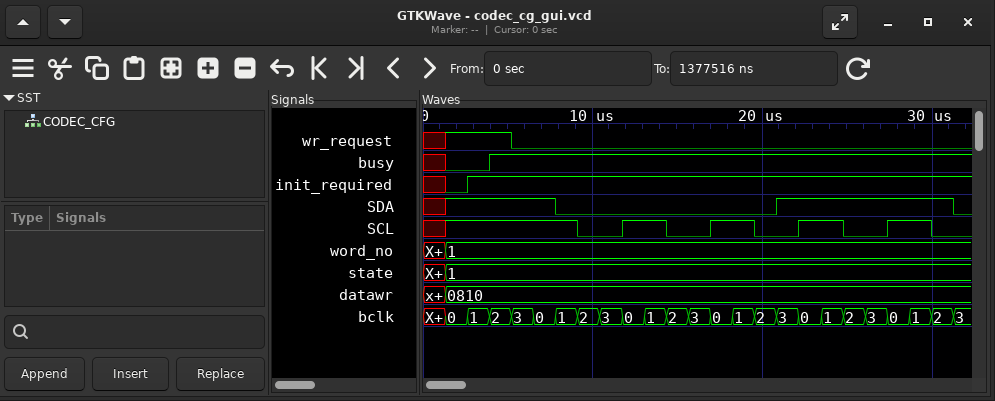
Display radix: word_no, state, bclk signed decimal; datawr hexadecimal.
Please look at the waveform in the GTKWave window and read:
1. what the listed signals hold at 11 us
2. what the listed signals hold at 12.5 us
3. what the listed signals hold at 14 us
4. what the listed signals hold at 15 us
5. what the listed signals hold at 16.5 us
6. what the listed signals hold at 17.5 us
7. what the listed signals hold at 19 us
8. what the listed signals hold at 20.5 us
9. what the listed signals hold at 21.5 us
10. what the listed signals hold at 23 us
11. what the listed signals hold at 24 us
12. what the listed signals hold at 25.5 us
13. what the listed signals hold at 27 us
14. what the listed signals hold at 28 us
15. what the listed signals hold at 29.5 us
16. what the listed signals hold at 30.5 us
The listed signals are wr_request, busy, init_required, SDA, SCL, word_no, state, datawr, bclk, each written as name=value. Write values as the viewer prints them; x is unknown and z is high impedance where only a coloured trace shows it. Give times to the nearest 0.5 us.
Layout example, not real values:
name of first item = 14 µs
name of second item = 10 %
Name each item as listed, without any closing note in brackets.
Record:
what the listed signals hold at 11 us = wr_request=0, busy=1, init_required=1, SDA=0, SCL=0, word_no=1, state=1, datawr=0810, bclk=3
what the listed signals hold at 12.5 us = wr_request=0, busy=1, init_required=1, SDA=0, SCL=1, word_no=1, state=1, datawr=0810, bclk=0
what the listed signals hold at 14 us = wr_request=0, busy=1, init_required=1, SDA=0, SCL=1, word_no=1, state=1, datawr=0810, bclk=1
what the listed signals hold at 15 us = wr_request=0, busy=1, init_required=1, SDA=0, SCL=0, word_no=1, state=1, datawr=0810, bclk=2
what the listed signals hold at 16.5 us = wr_request=0, busy=1, init_required=1, SDA=0, SCL=0, word_no=1, state=1, datawr=0810, bclk=3
what the listed signals hold at 17.5 us = wr_request=0, busy=1, init_required=1, SDA=0, SCL=1, word_no=1, state=1, datawr=0810, bclk=0
what the listed signals hold at 19 us = wr_request=0, busy=1, init_required=1, SDA=0, SCL=1, word_no=1, state=1, datawr=0810, bclk=1
what the listed signals hold at 20.5 us = wr_request=0, busy=1, init_required=1, SDA=0, SCL=0, word_no=1, state=1, datawr=0810, bclk=2
what the listed signals hold at 21.5 us = wr_request=0, busy=1, init_required=1, SDA=1, SCL=0, word_no=1, state=1, datawr=0810, bclk=3
what the listed signals hold at 23 us = wr_request=0, busy=1, init_required=1, SDA=1, SCL=1, word_no=1, state=1, datawr=0810, bclk=0
what the listed signals hold at 24 us = wr_request=0, busy=1, init_required=1, SDA=1, SCL=1, word_no=1, state=1, datawr=0810, bclk=1
what the listed signals hold at 25.5 us = wr_request=0, busy=1, init_required=1, SDA=1, SCL=0, word_no=1, state=1, datawr=0810, bclk=2
what the listed signals hold at 27 us = wr_request=0, busy=1, init_required=1, SDA=1, SCL=0, word_no=1, state=1, datawr=0810, bclk=3
what the listed signals hold at 28 us = wr_request=0, busy=1, init_required=1, SDA=1, SCL=1, word_no=1, state=1, datawr=0810, bclk=0
what the listed signals hold at 29.5 us = wr_request=0, busy=1, init_required=1, SDA=1, SCL=1, word_no=1, state=1, datawr=0810, bclk=1
what the listed signals hold at 30.5 us = wr_request=0, busy=1, init_required=1, SDA=1, SCL=0, word_no=1, state=1, datawr=0810, bclk=2
